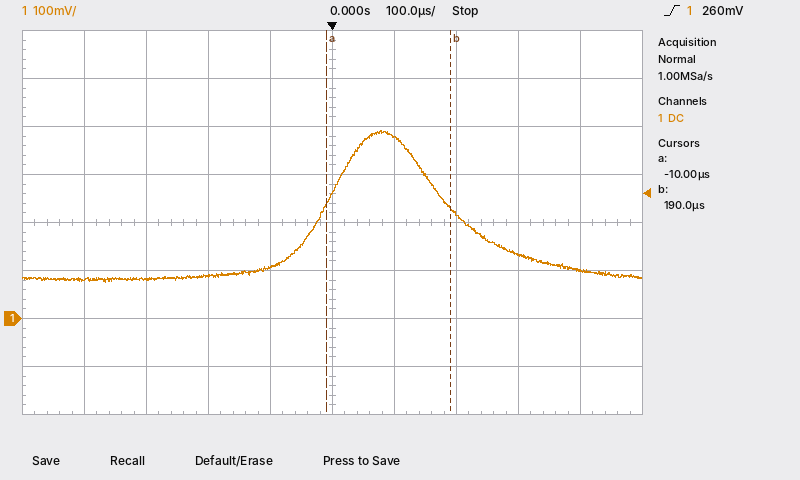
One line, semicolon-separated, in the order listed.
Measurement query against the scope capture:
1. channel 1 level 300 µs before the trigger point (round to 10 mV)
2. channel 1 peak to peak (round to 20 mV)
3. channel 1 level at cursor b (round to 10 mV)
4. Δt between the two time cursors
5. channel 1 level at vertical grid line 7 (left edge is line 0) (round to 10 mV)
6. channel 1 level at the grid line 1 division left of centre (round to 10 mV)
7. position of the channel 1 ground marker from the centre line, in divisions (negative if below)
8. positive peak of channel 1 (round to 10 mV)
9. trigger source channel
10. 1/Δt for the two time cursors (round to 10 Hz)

80 mV; 320 mV; 230 mV; 200 µs; 220 mV; 110 mV; -2.0 div; 390 mV; channel 1; 5.00 kHz
